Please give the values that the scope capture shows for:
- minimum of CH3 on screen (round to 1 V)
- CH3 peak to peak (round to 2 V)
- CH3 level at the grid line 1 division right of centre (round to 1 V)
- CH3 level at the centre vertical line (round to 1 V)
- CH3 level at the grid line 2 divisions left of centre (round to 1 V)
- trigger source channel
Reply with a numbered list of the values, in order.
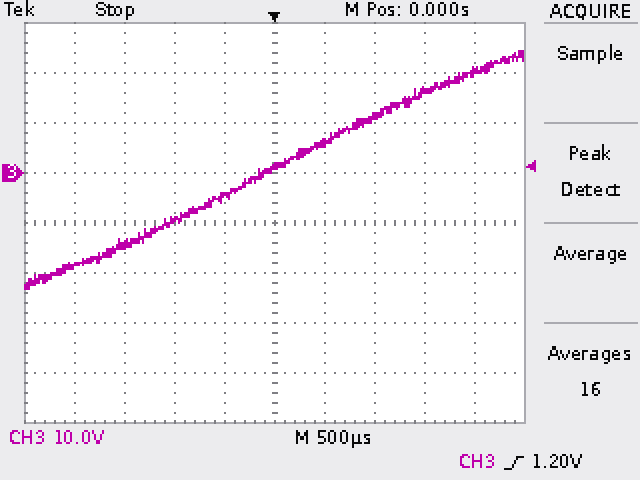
1. -23 V
2. 48 V
3. 6 V
4. 1 V
5. -9 V
6. CH3
